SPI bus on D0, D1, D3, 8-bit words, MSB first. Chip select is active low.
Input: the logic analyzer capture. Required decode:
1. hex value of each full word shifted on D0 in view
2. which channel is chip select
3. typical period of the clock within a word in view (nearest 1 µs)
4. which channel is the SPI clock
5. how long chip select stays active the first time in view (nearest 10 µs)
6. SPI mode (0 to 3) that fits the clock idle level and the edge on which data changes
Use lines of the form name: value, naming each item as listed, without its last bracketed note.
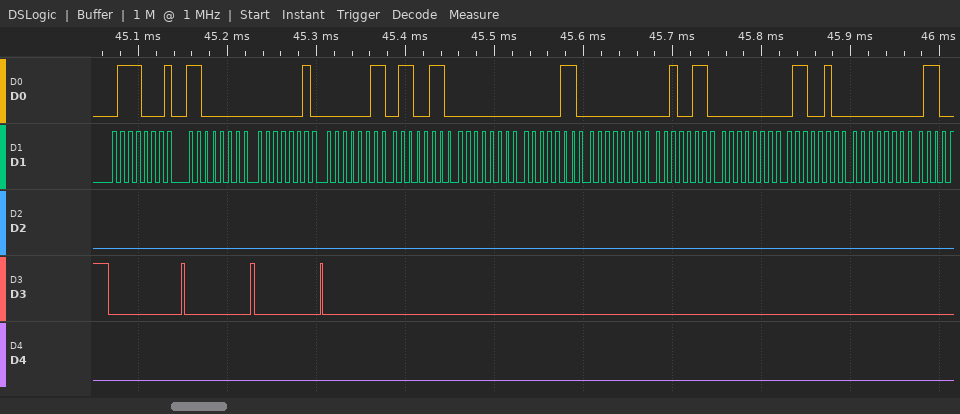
hex value of each full word shifted on D0 in view: 71, C0, 02, 03, 66, 00, 06, 00, 26, 00, 64, 00
which channel is chip select: D3
typical period of the clock within a word in view: 9 µs
which channel is the SPI clock: D1
how long chip select stays active the first time in view: 80 µs
SPI mode (0 to 3) that fits the clock idle level and the edge on which data changes: 0
